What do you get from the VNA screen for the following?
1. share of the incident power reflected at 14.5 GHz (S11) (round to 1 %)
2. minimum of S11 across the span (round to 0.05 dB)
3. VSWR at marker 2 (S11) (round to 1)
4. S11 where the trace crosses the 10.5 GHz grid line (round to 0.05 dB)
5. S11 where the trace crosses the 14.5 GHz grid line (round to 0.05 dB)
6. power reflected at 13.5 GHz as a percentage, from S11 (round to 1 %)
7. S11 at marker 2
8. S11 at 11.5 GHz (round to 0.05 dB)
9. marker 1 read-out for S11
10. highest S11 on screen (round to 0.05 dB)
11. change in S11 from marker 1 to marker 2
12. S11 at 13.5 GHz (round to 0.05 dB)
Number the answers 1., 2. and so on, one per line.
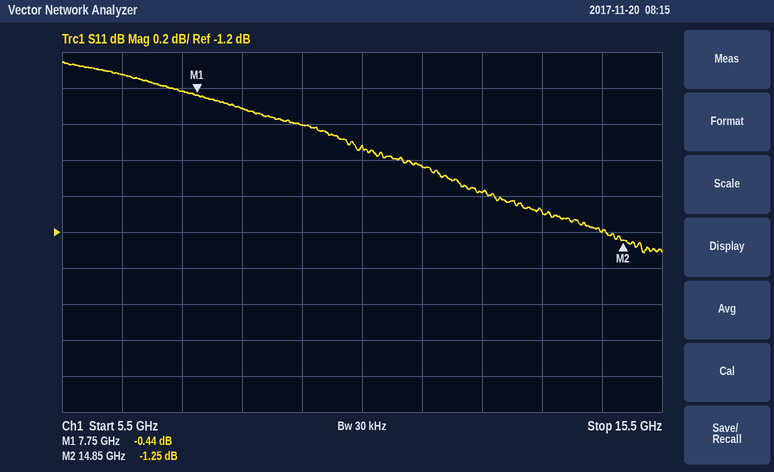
1. 76 %
2. -1.30 dB
3. 14
4. -0.70 dB
5. -1.20 dB
6. 78 %
7. -1.25 dB
8. -0.85 dB
9. -0.44 dB
10. -0.25 dB
11. -0.81 dB
12. -1.10 dB
